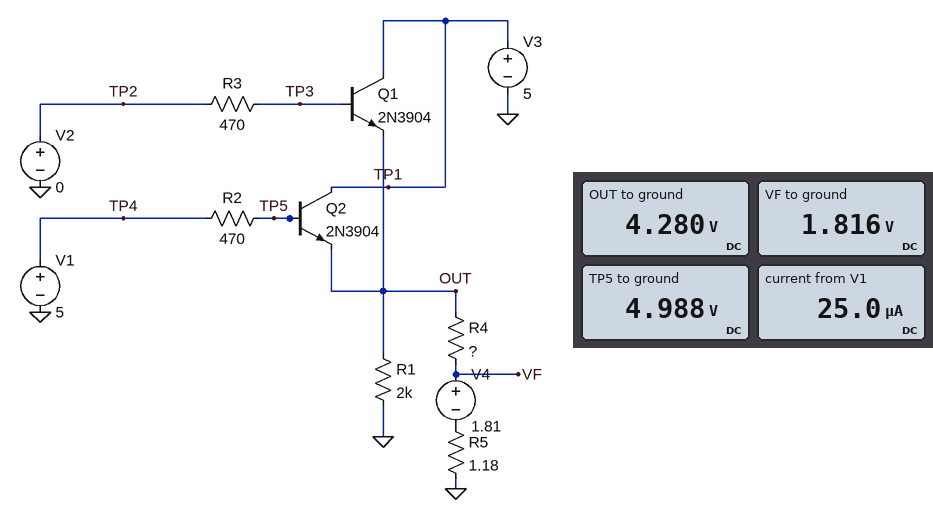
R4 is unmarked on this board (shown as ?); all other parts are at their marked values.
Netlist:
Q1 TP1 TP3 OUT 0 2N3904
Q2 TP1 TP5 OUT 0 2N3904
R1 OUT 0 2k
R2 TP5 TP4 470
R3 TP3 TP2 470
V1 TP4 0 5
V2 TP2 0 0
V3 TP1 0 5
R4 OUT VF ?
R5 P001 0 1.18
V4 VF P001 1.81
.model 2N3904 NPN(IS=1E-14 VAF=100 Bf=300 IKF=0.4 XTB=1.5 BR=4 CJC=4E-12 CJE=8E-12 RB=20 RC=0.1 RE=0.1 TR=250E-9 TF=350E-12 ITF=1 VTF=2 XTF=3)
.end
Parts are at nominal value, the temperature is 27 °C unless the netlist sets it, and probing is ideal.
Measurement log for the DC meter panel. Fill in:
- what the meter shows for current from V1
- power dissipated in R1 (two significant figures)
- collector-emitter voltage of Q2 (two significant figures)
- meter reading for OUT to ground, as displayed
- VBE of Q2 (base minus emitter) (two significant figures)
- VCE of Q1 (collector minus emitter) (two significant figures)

25.0 µA
9.2 mW
720 mV
4.280 V
710 mV
720 mV
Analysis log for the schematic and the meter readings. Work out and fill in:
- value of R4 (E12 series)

470 Ω
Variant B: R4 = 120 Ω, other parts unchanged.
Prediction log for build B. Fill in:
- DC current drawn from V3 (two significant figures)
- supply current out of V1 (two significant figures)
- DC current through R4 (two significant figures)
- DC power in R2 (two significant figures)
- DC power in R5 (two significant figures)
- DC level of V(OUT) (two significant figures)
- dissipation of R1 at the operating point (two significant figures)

22 mA
77 µA
20 mA
2.8 µW
470 µW
4.2 V
8.9 mW
